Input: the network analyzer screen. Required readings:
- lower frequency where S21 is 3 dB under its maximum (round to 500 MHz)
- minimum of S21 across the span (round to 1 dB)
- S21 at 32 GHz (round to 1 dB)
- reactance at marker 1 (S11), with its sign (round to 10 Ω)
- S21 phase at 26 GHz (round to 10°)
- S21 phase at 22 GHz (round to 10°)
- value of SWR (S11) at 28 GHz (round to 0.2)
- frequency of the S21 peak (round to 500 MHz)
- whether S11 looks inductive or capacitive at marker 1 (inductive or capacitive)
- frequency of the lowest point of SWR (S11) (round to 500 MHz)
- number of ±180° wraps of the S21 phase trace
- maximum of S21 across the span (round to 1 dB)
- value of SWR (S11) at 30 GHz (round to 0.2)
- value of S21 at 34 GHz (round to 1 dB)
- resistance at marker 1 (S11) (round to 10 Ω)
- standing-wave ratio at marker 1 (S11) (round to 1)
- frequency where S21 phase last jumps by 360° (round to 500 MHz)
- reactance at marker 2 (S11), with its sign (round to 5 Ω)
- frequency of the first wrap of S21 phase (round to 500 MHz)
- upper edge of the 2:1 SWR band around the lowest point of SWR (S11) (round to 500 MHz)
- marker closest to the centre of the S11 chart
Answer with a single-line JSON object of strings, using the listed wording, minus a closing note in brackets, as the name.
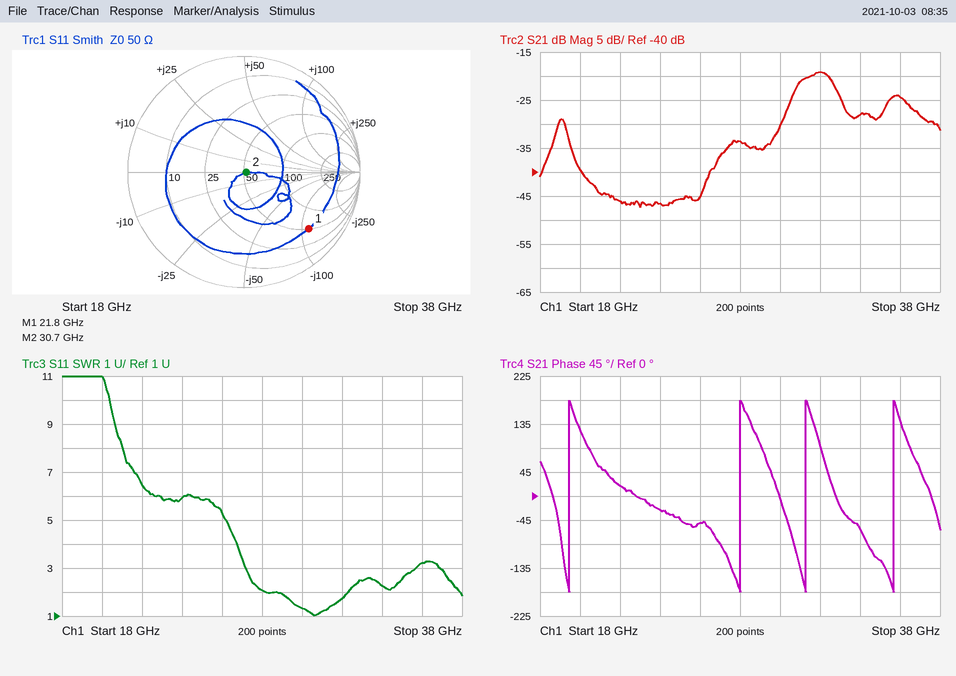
{"lower frequency where S21 is 3 dB under its maximum": "31.0 GHz", "minimum of S21 across the span": "-47 dB", "S21 at 32 GHz": "-19 dB", "reactance at marker 1 (S11), with its sign": "-110 Ω", "S21 phase at 26 GHz": "-50°", "S21 phase at 22 GHz": "20°", "value of SWR (S11) at 28 GHz": "2.0", "frequency of the S21 peak": "32.0 GHz", "whether S11 looks inductive or capacitive at marker 1": "capacitive", "frequency of the lowest point of SWR (S11)": "30.5 GHz", "number of ±180° wraps of the S21 phase trace": "4", "maximum of S21 across the span": "-19 dB", "value of SWR (S11) at 30 GHz": "1.4", "value of S21 at 34 GHz": "-28 dB", "resistance at marker 1 (S11)": "50 Ω", "standing-wave ratio at marker 1 (S11)": "7", "frequency where S21 phase last jumps by 360°": "35.5 GHz", "reactance at marker 2 (S11), with its sign": "0 Ω", "frequency of the first wrap of S21 phase": "19.5 GHz", "upper edge of the 2:1 SWR band around the lowest point of SWR (S11)": "32.5 GHz", "marker closest to the centre of the S11 chart": "marker 2"}
